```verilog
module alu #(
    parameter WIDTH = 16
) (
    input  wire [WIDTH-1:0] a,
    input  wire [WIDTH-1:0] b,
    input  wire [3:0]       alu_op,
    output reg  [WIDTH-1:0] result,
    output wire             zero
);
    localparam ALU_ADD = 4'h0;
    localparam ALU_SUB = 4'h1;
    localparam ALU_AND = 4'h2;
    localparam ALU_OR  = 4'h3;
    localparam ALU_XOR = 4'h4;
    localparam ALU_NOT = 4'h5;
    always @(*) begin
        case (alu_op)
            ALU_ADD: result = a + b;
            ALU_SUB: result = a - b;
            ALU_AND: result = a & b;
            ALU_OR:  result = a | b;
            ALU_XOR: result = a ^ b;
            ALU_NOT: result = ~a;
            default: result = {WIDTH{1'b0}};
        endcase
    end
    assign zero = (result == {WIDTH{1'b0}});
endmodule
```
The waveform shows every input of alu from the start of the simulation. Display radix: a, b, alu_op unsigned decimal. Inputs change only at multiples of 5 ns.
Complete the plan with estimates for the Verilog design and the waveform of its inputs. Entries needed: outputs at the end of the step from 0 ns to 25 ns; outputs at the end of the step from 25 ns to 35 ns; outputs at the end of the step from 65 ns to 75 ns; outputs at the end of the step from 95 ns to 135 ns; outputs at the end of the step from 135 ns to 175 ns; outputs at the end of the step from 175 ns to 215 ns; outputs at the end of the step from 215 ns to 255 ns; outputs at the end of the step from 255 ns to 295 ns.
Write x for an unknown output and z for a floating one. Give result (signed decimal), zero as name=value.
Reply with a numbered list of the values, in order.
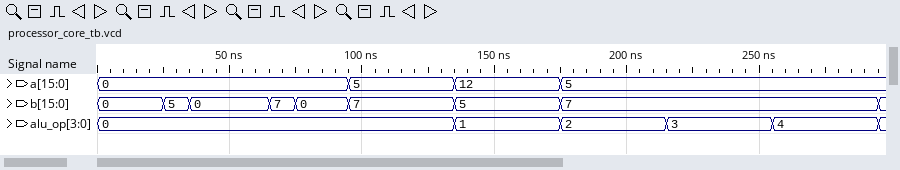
1. result=0, zero=1
2. result=5, zero=0
3. result=7, zero=0
4. result=12, zero=0
5. result=7, zero=0
6. result=5, zero=0
7. result=7, zero=0
8. result=2, zero=0
